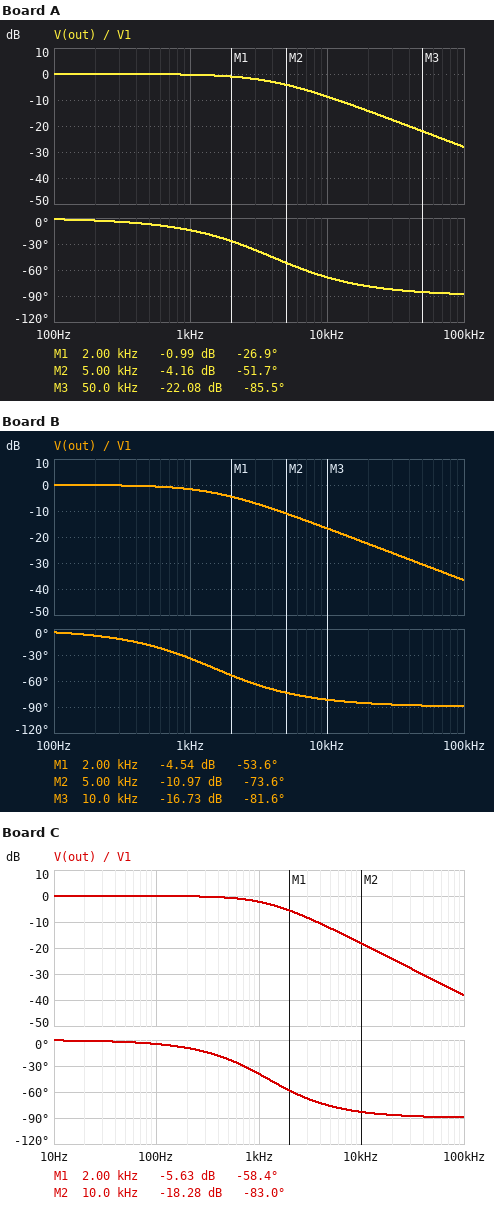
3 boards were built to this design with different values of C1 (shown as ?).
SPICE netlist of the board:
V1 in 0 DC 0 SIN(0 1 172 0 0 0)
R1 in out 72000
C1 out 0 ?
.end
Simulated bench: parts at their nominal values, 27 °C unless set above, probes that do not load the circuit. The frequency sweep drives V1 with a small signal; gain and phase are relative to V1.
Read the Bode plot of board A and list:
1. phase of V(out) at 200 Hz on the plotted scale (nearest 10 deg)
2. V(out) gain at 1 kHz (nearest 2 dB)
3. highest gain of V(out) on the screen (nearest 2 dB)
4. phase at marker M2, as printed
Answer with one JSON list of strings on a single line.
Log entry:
["0 deg", "0 dB", "0 dB", "-51.7 deg"]
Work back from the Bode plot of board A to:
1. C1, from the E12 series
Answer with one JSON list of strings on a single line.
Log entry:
["560 pF"]
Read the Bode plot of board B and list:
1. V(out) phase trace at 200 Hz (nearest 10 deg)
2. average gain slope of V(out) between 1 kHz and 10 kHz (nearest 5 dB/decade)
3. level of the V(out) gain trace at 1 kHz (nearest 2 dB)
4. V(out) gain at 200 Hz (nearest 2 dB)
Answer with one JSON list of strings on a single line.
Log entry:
["-10 deg", "-15 dB/decade", "-2 dB", "0 dB"]
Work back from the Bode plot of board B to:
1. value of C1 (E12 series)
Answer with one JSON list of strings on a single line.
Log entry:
["1.5 nF"]
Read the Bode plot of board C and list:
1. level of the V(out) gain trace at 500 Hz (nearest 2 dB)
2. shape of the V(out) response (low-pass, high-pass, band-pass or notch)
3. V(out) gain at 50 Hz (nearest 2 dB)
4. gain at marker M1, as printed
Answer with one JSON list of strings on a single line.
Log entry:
["0 dB", "low-pass", "0 dB", "-5.63 dB"]
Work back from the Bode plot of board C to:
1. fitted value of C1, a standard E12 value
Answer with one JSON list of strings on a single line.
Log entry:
["1.8 nF"]
